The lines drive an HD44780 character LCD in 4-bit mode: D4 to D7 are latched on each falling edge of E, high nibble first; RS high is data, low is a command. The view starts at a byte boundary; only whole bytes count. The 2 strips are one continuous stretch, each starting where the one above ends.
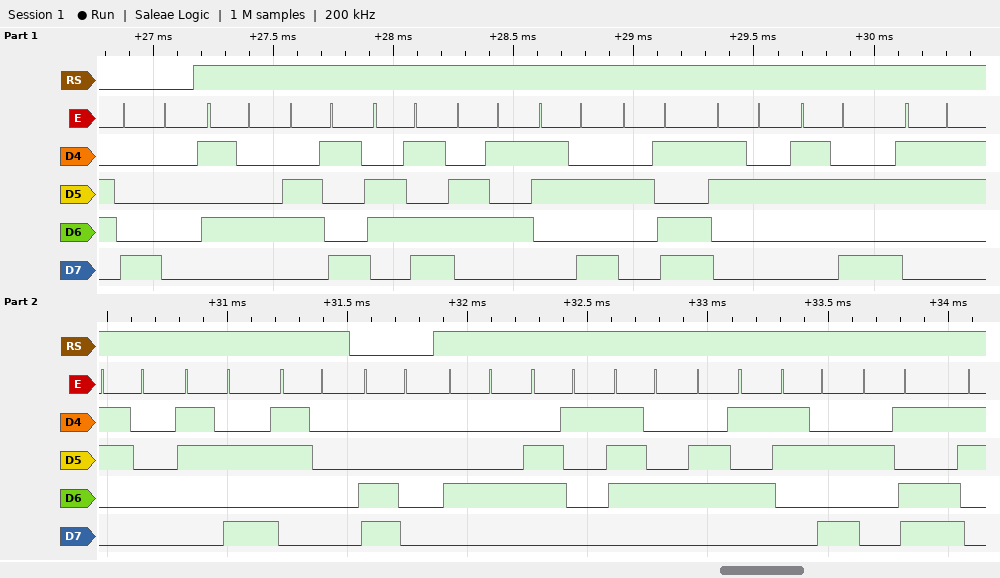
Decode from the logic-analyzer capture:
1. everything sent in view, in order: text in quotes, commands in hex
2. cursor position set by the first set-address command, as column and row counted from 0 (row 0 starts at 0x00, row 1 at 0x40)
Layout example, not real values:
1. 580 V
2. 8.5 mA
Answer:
1. 0x80 "Time:-2:30:0" 0xC0 "Date:-"
2. column 0, row 0
